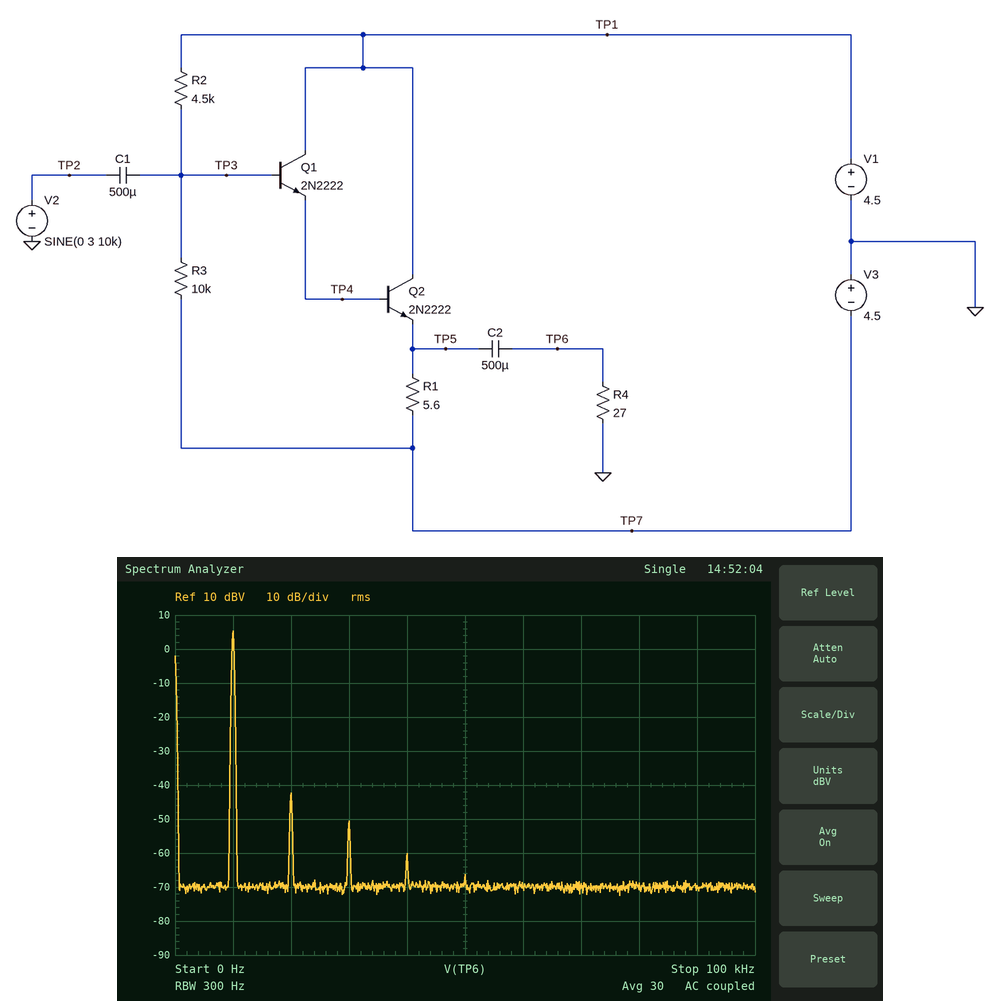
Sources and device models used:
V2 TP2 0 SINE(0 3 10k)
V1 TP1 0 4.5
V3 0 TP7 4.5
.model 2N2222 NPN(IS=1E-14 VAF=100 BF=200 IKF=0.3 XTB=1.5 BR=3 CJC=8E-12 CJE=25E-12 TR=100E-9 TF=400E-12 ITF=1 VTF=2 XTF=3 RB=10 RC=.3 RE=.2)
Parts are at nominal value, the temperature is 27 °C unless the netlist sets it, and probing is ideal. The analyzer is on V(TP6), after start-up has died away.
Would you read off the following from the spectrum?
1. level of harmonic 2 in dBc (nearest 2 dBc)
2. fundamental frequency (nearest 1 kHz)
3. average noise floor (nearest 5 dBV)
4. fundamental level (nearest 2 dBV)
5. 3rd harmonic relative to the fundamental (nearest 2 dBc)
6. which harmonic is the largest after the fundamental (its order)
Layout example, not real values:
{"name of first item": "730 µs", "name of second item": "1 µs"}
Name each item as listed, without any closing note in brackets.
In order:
{"level of harmonic 2 in dBc": "-48 dBc", "fundamental frequency": "10 kHz", "average noise floor": "-70 dBV", "fundamental level": "6 dBV", "3rd harmonic relative to the fundamental": "-56 dBc", "which harmonic is the largest after the fundamental": "2"}
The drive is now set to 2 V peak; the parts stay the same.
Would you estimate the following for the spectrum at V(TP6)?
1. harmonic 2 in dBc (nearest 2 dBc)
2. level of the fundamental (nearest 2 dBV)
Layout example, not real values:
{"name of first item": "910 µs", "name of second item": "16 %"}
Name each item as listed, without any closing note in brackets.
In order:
{"harmonic 2 in dBc": "-50 dBc", "level of the fundamental": "2 dBV"}
